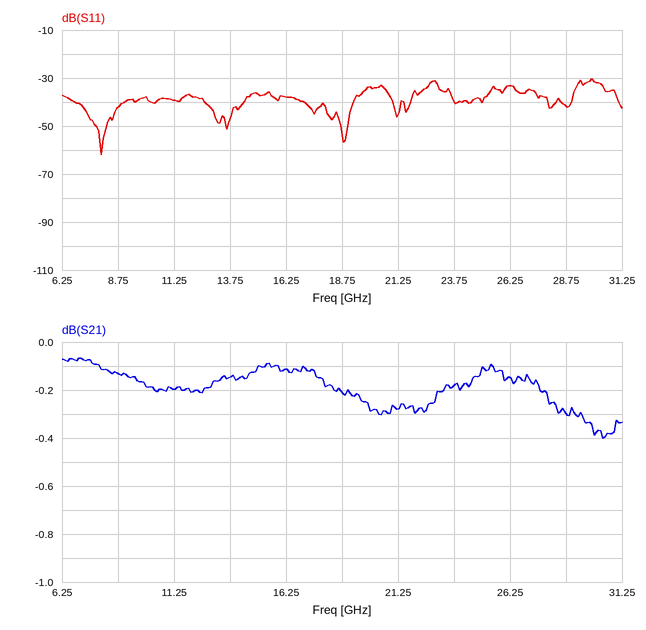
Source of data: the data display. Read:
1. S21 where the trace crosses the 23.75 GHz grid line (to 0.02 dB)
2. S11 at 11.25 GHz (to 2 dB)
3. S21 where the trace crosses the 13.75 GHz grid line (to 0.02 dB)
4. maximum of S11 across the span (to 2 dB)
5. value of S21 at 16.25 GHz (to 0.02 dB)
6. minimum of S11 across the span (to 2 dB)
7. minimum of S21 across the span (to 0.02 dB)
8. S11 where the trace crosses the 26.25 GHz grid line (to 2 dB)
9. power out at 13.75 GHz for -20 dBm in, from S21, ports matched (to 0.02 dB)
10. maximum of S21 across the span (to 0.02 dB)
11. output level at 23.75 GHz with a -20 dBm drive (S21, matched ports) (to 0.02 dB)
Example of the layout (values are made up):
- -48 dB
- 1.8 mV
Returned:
- -0.18 dB
- -40 dB
- -0.14 dB
- -30 dB
- -0.12 dB
- -62 dB
- -0.40 dB
- -34 dB
- -20.14 dBm
- -0.06 dB
- -20.18 dBm
